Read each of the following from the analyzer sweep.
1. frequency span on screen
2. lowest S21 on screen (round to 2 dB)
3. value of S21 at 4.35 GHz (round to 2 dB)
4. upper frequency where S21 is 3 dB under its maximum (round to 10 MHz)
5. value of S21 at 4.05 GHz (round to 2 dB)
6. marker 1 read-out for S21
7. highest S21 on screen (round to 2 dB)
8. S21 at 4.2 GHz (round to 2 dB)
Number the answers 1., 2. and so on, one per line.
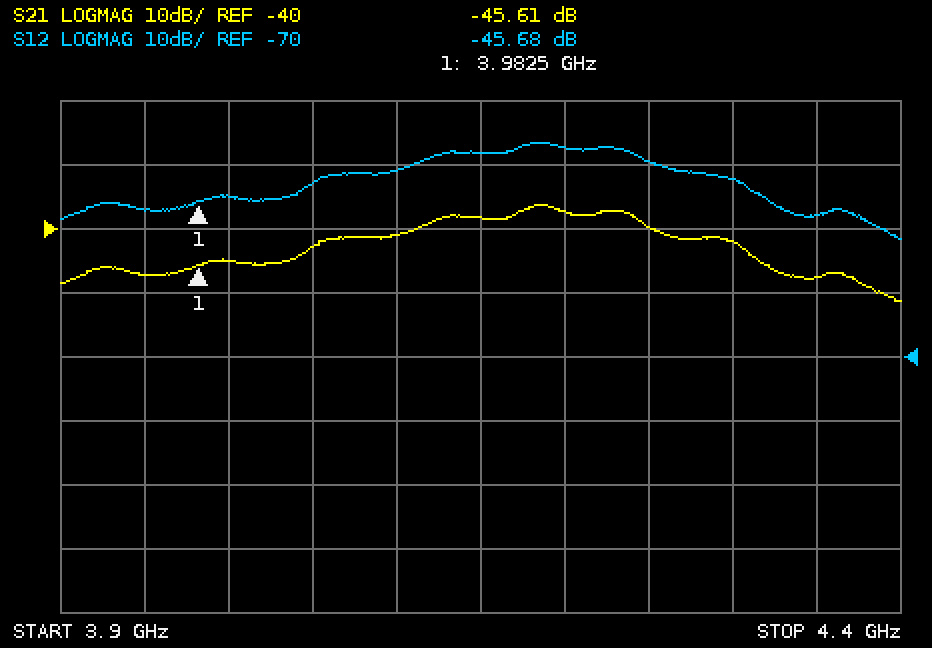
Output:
1. 500 MHz
2. -52 dB
3. -48 dB
4. 4.25 GHz
5. -42 dB
6. -45.61 dB
7. -36 dB
8. -38 dB
